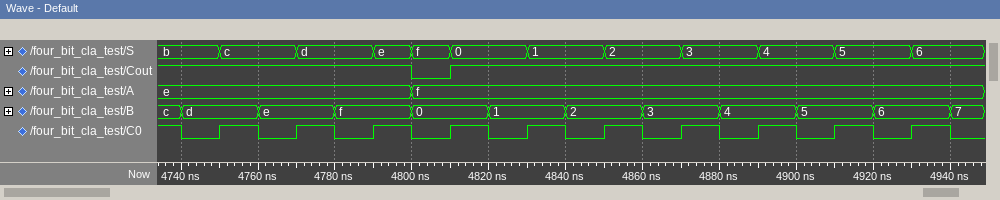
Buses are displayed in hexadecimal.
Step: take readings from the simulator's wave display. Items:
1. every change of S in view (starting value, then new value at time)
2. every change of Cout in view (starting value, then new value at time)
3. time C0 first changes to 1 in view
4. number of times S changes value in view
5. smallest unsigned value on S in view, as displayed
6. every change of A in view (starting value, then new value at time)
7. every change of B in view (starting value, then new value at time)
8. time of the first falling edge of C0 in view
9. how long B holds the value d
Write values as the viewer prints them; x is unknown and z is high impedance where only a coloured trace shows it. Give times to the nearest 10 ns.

b, c at 4750 ns, d at 4770 ns, e at 4790 ns, f at 4800 ns, 0 at 4810 ns, 1 at 4830 ns, 2 at 4850 ns, 3 at 4870 ns, 4 at 4890 ns, 5 at 4910 ns, 6 at 4930 ns
1, 0 at 4800 ns, 1 at 4810 ns
4750 ns
11
0
e, f at 4800 ns
c, d at 4740 ns, e at 4760 ns, f at 4780 ns, 0 at 4800 ns, 1 at 4820 ns, 2 at 4840 ns, 3 at 4860 ns, 4 at 4880 ns, 5 at 4900 ns, 6 at 4920 ns, 7 at 4940 ns
4740 ns
20 ns
